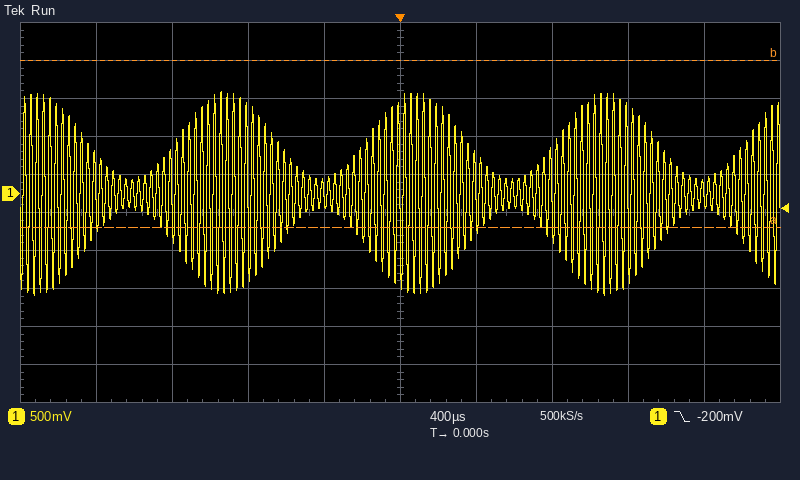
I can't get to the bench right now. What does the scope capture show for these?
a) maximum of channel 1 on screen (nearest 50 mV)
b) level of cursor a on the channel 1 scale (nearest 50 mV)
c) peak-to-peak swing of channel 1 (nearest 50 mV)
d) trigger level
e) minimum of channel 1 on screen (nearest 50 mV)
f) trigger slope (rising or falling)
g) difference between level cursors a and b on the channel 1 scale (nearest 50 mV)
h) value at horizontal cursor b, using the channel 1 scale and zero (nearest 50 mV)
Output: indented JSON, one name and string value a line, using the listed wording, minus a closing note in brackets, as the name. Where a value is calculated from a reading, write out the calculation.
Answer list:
{
  "maximum of channel 1 on screen": "1.35 V",
  "level of cursor a on the channel 1 scale": "-450 mV",
  "peak-to-peak swing of channel 1": "1.35 V − (-1.35 V) = 2.70 V",
  "trigger level": "-200 mV",
  "minimum of channel 1 on screen": "-1.35 V",
  "trigger slope": "falling",
  "difference between level cursors a and b on the channel 1 scale": "2.20 V",
  "value at horizontal cursor b, using the channel 1 scale and zero": "1.75 V"
}
